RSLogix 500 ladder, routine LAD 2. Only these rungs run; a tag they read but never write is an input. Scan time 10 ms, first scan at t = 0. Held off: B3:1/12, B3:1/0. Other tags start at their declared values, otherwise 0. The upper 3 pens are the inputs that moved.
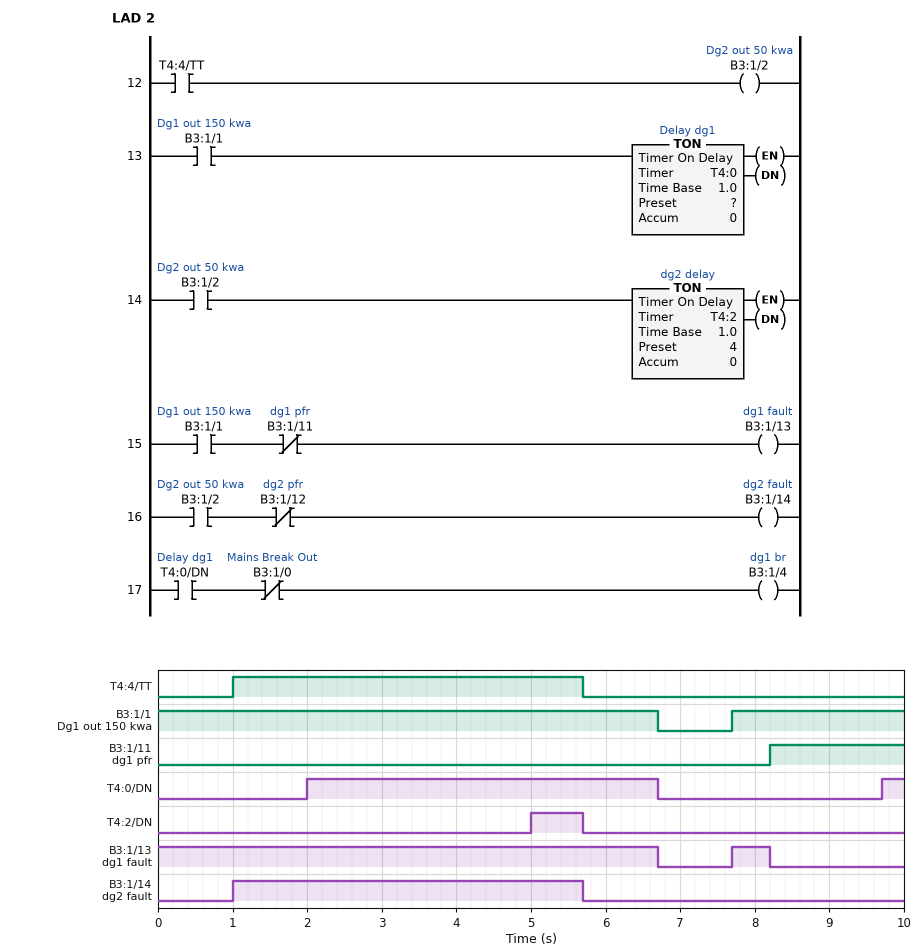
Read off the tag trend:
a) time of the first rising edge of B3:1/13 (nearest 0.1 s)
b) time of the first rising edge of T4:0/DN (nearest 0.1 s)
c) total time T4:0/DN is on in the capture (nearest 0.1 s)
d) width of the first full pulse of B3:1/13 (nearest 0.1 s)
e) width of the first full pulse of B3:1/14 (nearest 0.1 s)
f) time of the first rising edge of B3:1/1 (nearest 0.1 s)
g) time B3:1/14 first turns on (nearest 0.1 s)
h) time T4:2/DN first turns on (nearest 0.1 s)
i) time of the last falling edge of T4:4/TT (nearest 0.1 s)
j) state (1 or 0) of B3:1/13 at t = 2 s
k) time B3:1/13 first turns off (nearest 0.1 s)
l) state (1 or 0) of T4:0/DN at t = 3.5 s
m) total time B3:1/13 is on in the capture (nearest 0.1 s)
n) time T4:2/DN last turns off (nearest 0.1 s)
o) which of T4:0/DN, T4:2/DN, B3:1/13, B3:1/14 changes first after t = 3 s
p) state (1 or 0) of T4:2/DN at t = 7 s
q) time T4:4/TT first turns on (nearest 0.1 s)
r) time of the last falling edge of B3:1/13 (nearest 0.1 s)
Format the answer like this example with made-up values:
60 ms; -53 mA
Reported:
7.7 s; 2.0 s; 5.0 s; 0.5 s; 4.7 s; 7.7 s; 1.0 s; 5.0 s; 5.7 s; 1; 6.7 s; 1; 7.2 s; 5.7 s; T4:2/DN; 0; 1.0 s; 8.2 s
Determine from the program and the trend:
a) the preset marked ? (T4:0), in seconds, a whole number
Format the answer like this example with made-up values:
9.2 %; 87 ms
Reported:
2 s
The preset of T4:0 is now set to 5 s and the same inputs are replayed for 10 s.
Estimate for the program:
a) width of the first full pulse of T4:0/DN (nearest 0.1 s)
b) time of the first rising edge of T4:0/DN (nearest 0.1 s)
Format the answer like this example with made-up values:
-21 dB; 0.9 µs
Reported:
1.7 s; 5.0 s
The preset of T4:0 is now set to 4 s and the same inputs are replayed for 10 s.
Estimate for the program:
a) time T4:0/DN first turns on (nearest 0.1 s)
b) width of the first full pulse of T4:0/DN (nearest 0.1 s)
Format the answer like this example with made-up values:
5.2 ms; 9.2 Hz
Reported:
4.0 s; 2.7 s
